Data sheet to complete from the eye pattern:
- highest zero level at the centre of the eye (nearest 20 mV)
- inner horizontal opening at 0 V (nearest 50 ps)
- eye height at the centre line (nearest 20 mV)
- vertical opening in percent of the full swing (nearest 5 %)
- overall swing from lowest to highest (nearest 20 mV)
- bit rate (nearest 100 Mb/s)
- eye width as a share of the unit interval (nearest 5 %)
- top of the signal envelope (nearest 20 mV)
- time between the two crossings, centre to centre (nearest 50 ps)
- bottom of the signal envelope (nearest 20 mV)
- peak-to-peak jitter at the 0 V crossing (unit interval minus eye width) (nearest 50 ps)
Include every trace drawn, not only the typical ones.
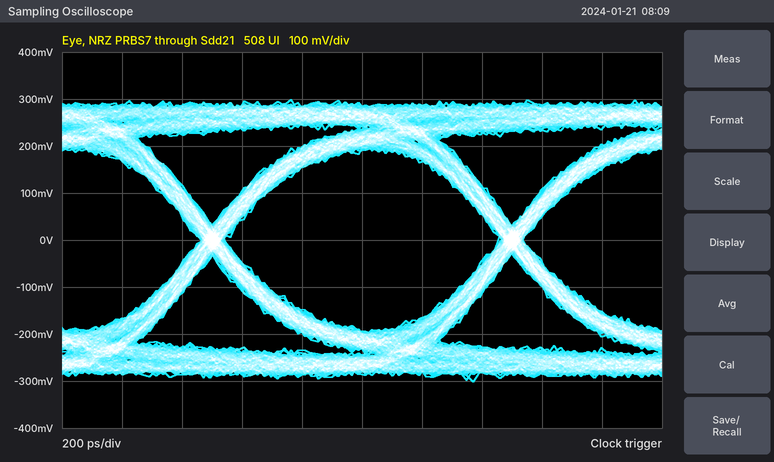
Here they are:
-200 mV
900 ps
380 mV
65 %
600 mV
1.0 Gb/s
90 %
300 mV
1.00 ns
-300 mV
100 ps
